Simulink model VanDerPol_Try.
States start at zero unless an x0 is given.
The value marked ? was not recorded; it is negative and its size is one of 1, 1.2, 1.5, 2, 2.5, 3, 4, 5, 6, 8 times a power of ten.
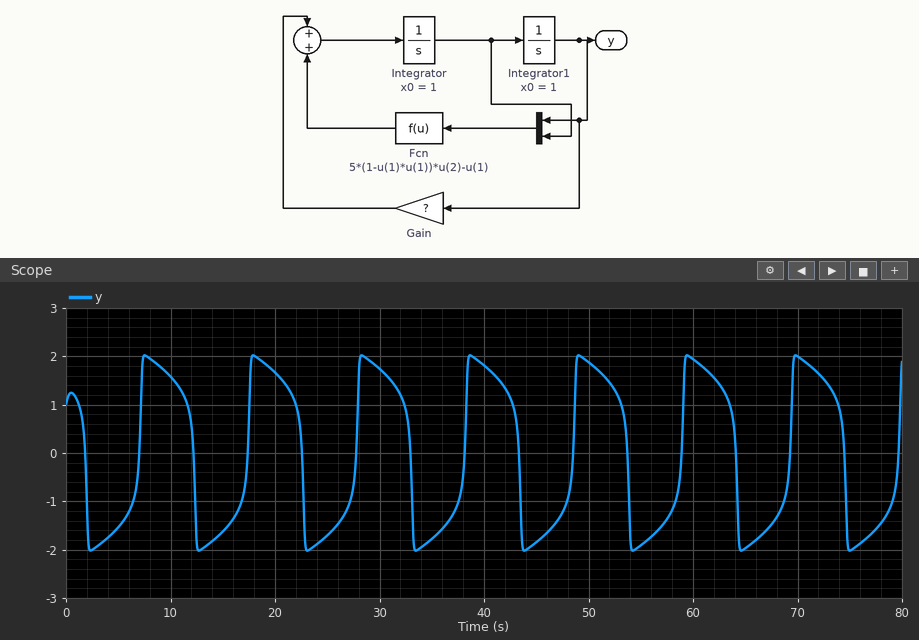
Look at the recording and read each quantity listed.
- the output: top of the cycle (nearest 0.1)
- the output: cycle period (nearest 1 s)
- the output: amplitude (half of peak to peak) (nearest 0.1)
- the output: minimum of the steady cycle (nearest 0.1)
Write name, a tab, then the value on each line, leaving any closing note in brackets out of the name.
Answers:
the output: top of the cycle	2.0
the output: cycle period	10 s
the output: amplitude (half of peak to peak)	2.0
the output: minimum of the steady cycle	-2.0
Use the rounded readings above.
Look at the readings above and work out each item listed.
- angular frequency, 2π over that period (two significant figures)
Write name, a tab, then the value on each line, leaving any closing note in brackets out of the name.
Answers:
angular frequency, 2π over that period	0.63 rad/s
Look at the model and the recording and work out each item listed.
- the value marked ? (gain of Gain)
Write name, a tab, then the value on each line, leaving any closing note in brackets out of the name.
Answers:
the value marked ?	-0.15
